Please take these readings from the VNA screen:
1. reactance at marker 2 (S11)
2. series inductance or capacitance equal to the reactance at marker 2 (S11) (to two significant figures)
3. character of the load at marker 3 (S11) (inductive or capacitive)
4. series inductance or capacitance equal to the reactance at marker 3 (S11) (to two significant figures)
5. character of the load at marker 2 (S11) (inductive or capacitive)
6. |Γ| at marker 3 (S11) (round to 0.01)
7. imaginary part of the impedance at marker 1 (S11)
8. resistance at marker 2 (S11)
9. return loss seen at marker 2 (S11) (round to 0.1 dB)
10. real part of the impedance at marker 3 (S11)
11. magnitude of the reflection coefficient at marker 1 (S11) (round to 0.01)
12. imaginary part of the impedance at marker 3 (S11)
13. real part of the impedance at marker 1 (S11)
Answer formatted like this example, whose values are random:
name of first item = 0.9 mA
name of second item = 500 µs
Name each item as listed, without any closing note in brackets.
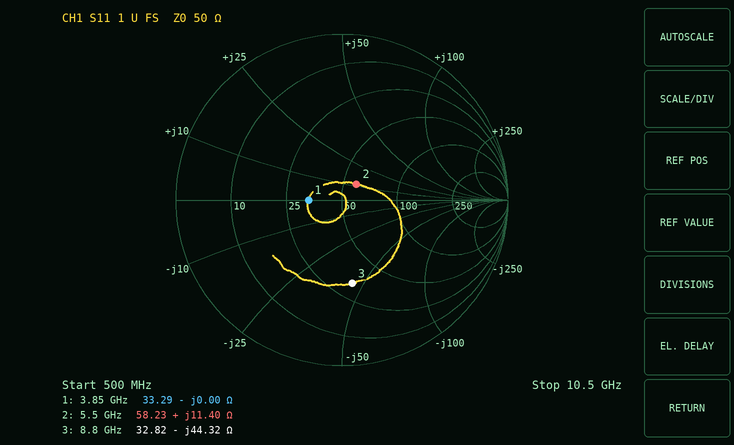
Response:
reactance at marker 2 = +11.40 Ω
series inductance or capacitance equal to the reactance at marker 2 (S11) = 330 pH
character of the load at marker 3 (S11) = capacitive
series inductance or capacitance equal to the reactance at marker 3 (S11) = 410 fF
character of the load at marker 2 (S11) = inductive
|Γ| at marker 3 (S11) = 0.51
imaginary part of the impedance at marker 1 = -0.00 Ω
resistance at marker 2 = 58.23 Ω
return loss seen at marker 2 (S11) = 17.8 dB
real part of the impedance at marker 3 = 32.82 Ω
magnitude of the reflection coefficient at marker 1 (S11) = 0.20
imaginary part of the impedance at marker 3 = -44.32 Ω
real part of the impedance at marker 1 = 33.29 Ω
